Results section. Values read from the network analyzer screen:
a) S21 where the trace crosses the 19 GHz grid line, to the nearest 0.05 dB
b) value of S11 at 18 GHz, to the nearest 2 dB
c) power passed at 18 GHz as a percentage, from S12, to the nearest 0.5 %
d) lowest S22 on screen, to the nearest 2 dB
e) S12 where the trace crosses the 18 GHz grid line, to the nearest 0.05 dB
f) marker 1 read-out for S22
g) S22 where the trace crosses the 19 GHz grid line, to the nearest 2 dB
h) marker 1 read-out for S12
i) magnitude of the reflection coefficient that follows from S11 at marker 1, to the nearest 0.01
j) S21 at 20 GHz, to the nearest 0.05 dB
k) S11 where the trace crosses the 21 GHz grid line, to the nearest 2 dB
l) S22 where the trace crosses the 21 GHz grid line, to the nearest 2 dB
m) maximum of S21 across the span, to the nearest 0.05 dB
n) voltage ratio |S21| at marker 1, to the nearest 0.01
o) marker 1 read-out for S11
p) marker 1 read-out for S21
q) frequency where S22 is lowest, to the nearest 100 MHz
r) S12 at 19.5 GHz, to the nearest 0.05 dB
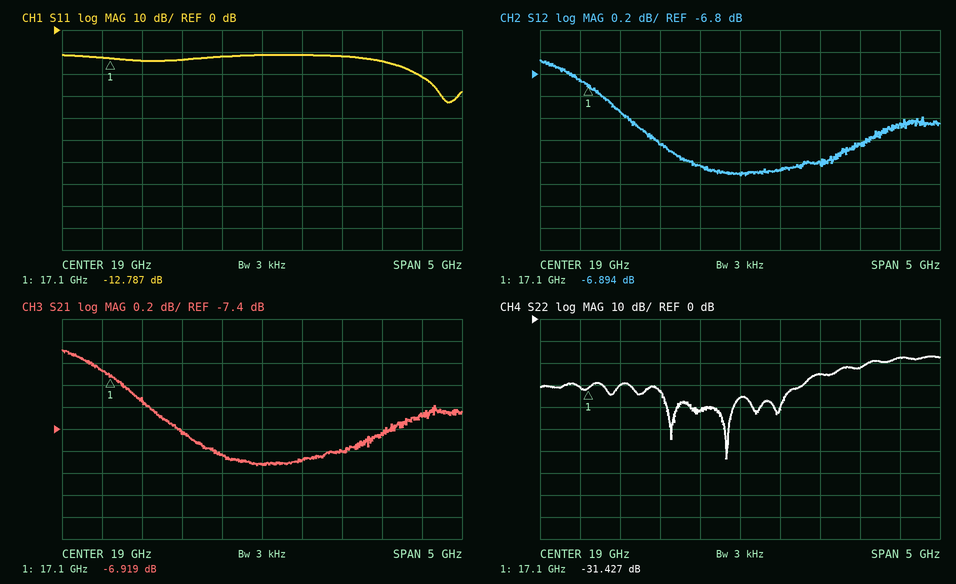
-7.70 dB
-14 dB
18.0 %
-64 dB
-7.45 dB
-31.427 dB
-36 dB
-6.894 dB
0.23
-7.60 dB
-22 dB
-18 dB
-6.70 dB
0.45
-12.787 dB
-6.919 dB
18.8 GHz
-7.65 dB
